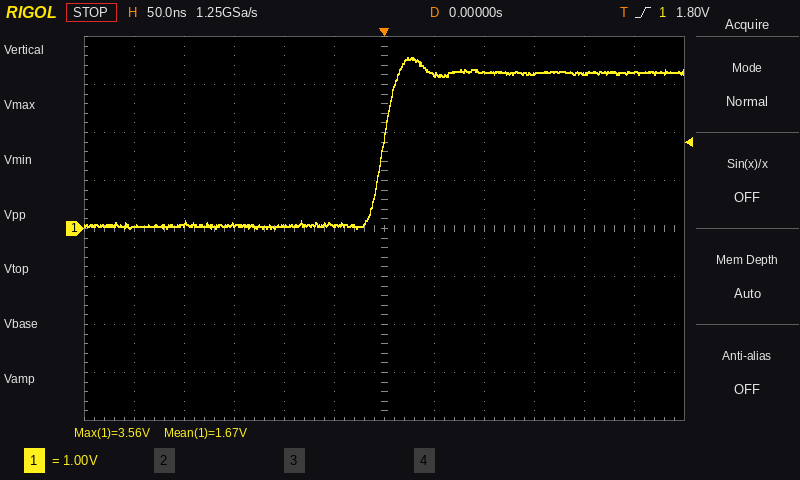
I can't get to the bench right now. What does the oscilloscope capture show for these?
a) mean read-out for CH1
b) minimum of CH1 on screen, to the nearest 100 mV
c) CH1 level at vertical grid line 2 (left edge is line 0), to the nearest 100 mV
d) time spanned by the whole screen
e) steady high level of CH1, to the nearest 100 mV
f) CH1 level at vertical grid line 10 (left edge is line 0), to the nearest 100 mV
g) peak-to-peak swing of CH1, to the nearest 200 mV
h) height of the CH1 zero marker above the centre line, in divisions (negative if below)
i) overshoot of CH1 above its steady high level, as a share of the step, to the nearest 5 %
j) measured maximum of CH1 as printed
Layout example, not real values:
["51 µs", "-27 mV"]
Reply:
["1.67 V", "0.0 V", "100 mV", "600 ns", "3.2 V", "3.2 V", "3.6 V", "0.0 div", "10 %", "3.56 V"]
